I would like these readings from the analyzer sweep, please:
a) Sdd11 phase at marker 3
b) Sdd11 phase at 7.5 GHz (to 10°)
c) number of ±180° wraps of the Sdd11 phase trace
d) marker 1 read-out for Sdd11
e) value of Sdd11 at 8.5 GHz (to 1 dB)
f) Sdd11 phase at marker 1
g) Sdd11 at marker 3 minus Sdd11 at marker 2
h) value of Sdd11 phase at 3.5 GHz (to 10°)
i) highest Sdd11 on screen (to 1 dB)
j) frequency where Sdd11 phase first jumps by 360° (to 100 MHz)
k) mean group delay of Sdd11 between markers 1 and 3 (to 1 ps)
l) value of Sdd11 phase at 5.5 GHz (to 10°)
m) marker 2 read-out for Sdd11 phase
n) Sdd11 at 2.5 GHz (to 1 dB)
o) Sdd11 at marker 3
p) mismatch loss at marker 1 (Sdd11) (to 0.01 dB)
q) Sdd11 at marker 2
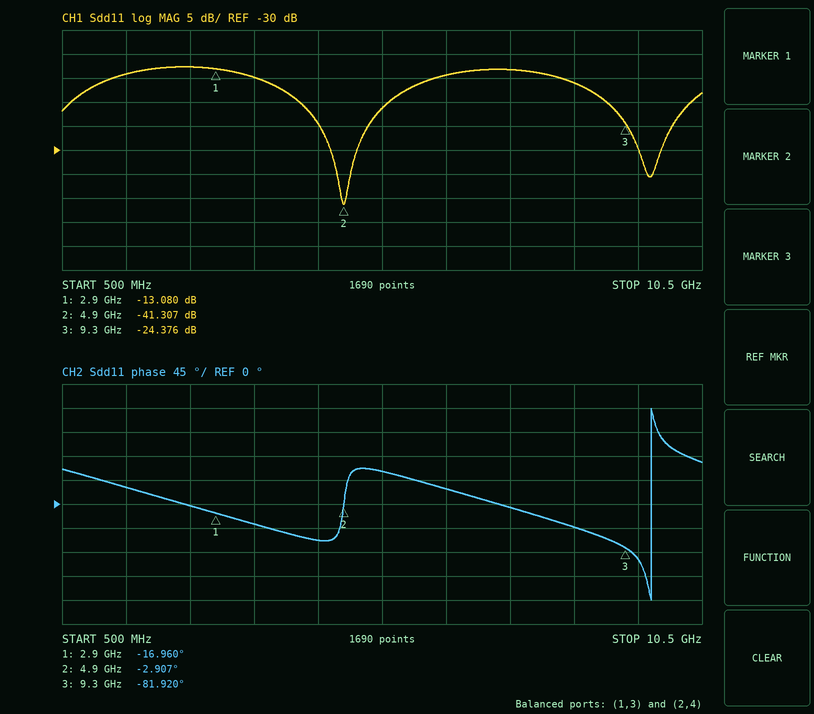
-81.920°
-10°
1
-13.080 dB
-16 dB
-16.960°
16.931 dB
-40°
-13 dB
9.7 GHz
28 ps
60°
-2.907°
-13 dB
-24.376 dB
0.22 dB
-41.307 dB
